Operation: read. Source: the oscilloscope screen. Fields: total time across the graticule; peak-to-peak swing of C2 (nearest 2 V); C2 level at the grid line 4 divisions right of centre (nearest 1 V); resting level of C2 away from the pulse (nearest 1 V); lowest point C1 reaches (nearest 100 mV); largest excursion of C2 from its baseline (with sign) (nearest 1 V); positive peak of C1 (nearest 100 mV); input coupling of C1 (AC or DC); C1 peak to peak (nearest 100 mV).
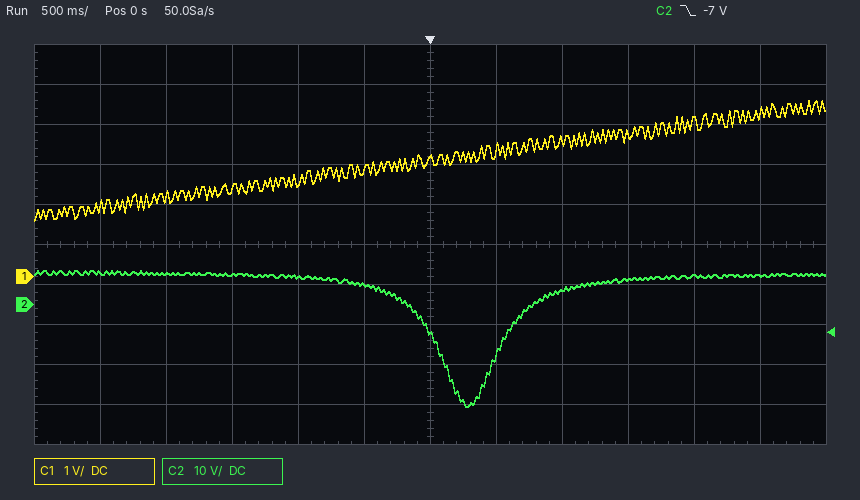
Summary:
6 s
34 V
7 V
7 V
1.4 V
-33 V
4.4 V
DC
3.0 V
